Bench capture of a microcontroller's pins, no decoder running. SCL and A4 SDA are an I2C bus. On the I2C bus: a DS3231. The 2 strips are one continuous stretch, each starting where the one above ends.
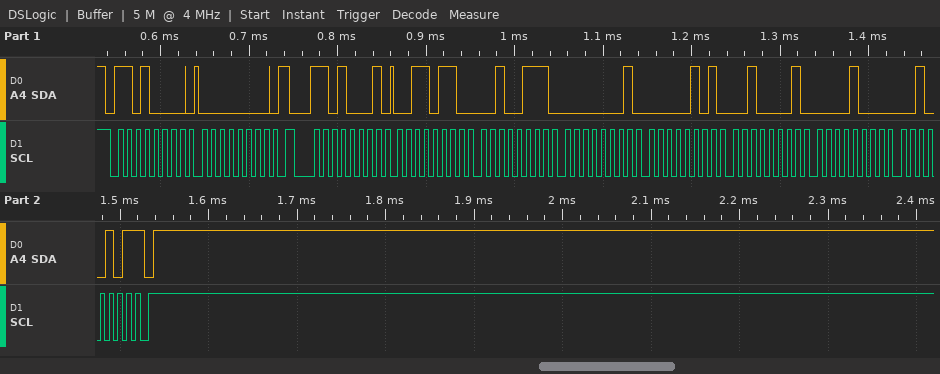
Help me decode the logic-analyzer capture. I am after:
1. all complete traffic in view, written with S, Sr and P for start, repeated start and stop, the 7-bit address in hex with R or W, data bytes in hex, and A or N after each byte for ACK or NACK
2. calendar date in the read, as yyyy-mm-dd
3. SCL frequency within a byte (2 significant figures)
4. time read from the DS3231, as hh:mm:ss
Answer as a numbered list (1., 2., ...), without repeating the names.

1. S 68W A 00 A Sr 68R A 36 A 27 A 01 A 05 A 21 A 08 A 25 N P
2. 2025-08-21
3. 100 kHz
4. 01:27:36
